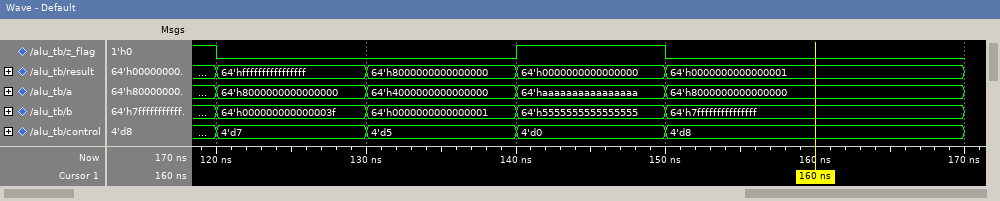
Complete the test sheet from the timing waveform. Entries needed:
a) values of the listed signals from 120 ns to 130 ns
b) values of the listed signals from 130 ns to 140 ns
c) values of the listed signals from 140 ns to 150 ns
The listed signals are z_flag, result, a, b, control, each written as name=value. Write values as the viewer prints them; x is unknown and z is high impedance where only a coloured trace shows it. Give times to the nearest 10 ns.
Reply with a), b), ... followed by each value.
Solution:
a) z_flag=0, result=64'hffffffffffffffff, a=64'h8000000000000000, b=64'h000000000000003f, control=4'd7
b) z_flag=0, result=64'h8000000000000000, a=64'h4000000000000000, b=64'h0000000000000001, control=4'd5
c) z_flag=1, result=64'h0000000000000000, a=64'haaaaaaaaaaaaaaaa, b=64'h5555555555555555, control=4'd0
